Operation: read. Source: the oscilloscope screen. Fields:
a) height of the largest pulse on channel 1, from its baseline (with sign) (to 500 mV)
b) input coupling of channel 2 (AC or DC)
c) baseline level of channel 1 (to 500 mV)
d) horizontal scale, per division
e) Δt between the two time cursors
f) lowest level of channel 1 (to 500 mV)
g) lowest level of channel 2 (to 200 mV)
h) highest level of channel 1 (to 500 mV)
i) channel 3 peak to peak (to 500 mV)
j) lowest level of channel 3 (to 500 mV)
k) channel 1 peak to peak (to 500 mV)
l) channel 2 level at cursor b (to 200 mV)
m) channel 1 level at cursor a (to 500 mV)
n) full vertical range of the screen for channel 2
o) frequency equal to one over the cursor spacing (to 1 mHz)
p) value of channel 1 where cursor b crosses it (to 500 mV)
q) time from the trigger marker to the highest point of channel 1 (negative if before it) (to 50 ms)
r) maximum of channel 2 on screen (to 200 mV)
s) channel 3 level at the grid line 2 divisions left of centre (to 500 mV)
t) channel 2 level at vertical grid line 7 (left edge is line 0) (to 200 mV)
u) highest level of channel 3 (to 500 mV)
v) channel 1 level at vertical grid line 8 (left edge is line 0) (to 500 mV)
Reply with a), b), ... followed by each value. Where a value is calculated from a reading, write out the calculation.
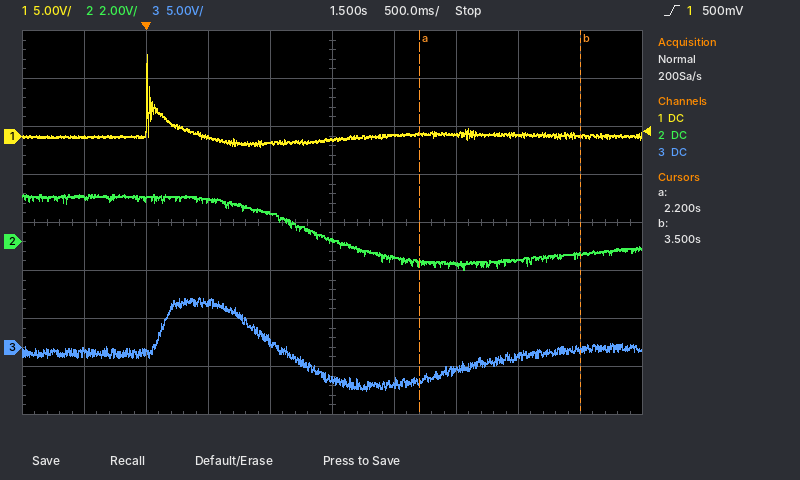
a) 8.5 V − (0.0 V) = +8.5 V
b) DC
c) 0.0 V
d) 500 ms
e) 3.5 s − (2.2 s) = 1.30 s
f) -1.0 V
g) -1.2 V
h) 8.5 V
i) 5.0 V − (-4.5 V) = 9.5 V
j) -4.5 V
k) 8.5 V − (-1.0 V) = 9.5 V
l) -600 mV
m) 0.0 V
n) 16 V
o) 1 / 1.30 s ≈ 769 mHz
p) 0.0 V
q) 0 ms
r) 2.0 V
s) 4.5 V
t) -1.0 V
u) 5.0 V
v) 0.0 V
